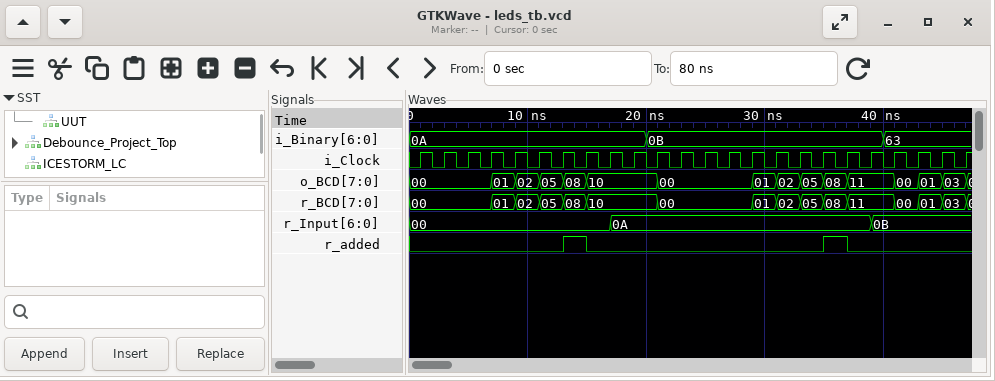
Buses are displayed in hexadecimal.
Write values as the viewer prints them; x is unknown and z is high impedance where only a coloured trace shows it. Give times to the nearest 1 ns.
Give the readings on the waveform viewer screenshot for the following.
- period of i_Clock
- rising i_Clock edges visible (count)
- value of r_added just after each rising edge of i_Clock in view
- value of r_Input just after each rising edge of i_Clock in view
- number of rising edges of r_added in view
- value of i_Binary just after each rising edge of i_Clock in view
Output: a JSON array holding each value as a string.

["2 ns", "24", "0 0 0 0 0 0 1 0 0 0 0 0 0 0 0 0 0 1 0 0 0 0 0 0", "00, 00, 00, 00, 00, 00, 00, 00, 0A, 0A, 0A, 0A, 0A, 0A, 0A, 0A, 0A, 0A, 0A, 0B, 0B, 0B, 0B, 0B", "2", "0A, 0A, 0A, 0A, 0A, 0A, 0A, 0A, 0A, 0A, 0B, 0B, 0B, 0B, 0B, 0B, 0B, 0B, 0B, 0B, 63, 63, 63, 63"]
